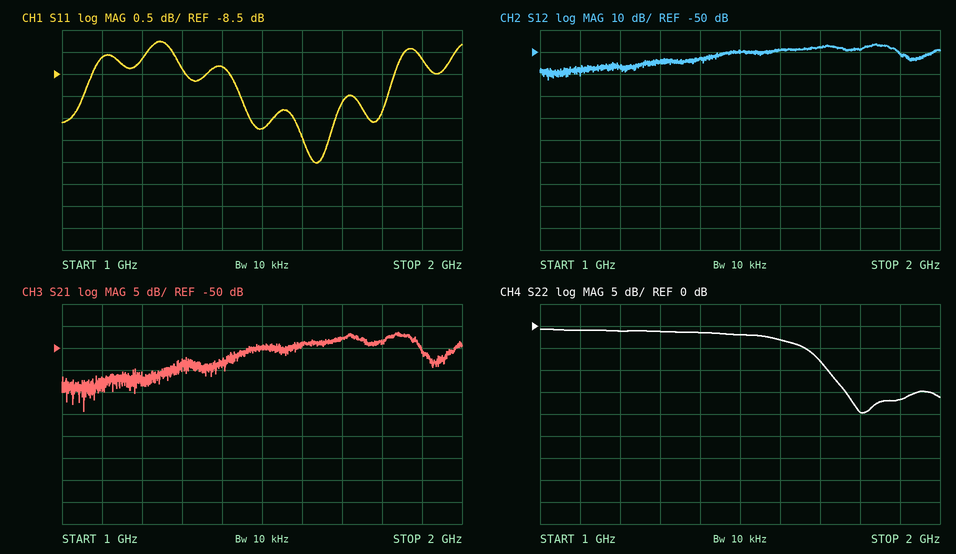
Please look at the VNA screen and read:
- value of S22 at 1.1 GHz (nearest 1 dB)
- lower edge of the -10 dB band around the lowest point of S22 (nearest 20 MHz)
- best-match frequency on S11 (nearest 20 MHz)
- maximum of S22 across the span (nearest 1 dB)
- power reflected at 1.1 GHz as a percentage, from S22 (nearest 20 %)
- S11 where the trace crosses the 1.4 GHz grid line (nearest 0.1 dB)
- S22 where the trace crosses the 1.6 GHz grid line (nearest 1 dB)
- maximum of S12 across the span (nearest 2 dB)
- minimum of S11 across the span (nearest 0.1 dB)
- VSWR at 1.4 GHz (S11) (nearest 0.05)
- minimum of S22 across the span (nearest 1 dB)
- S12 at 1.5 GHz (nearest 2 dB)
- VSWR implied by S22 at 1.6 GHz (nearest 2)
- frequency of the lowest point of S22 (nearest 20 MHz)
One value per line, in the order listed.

-1 dB
1.72 GHz
1.64 GHz
-1 dB
80 %
-8.3 dB
-3 dB
-46 dB
-10.5 dB
2.25
-20 dB
-50 dB
6
1.80 GHz
